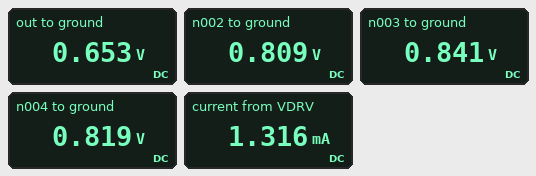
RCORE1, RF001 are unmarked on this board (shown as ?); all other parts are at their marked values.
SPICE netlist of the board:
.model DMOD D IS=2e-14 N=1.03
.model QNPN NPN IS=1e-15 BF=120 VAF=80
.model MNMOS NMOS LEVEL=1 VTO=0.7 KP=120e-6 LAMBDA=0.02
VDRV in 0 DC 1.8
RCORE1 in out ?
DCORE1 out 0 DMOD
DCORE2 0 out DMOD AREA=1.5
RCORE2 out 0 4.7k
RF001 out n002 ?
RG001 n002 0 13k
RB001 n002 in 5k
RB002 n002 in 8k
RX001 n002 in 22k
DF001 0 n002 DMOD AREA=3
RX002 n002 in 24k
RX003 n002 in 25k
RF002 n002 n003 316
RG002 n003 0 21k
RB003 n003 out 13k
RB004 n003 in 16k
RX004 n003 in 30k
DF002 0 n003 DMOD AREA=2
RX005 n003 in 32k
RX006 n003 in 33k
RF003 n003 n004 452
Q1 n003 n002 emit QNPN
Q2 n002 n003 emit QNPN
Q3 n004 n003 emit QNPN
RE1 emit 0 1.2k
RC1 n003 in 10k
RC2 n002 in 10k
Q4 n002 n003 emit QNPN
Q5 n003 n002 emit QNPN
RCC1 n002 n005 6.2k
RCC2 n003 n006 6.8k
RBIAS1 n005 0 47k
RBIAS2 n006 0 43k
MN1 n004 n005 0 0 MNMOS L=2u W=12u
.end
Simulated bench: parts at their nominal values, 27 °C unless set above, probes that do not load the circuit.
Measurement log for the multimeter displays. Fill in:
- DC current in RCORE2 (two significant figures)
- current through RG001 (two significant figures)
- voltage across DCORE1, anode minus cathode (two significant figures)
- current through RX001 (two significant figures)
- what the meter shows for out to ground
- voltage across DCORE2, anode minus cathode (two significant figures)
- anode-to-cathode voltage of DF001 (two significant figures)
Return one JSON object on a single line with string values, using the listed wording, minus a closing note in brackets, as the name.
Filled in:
{"DC current in RCORE2": "140 µA", "current through RG001": "62 µA", "voltage across DCORE1, anode minus cathode": "650 mV", "current through RX001": "45 µA", "what the meter shows for out to ground": "0.653 V", "voltage across DCORE2, anode minus cathode": "-650 mV", "anode-to-cathode voltage of DF001": "-810 mV"}
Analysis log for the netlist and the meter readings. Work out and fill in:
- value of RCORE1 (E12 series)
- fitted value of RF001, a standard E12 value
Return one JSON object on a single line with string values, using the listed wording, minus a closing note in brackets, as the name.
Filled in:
{"value of RCORE1": "2.2 kΩ", "fitted value of RF001, a standard E12 value": "330 Ω"}
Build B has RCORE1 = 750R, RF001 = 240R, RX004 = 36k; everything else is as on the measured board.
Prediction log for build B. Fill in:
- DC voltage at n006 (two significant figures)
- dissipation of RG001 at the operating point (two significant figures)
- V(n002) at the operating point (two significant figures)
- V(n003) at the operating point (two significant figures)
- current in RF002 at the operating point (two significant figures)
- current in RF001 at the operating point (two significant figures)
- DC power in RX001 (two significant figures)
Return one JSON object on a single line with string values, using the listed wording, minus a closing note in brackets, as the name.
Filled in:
{"DC voltage at n006": "710 mV", "dissipation of RG001 at the operating point": "48 µW", "V(n002) at the operating point": "790 mV", "V(n003) at the operating point": "830 mV", "current in RF002 at the operating point": "110 µA", "current in RF001 at the operating point": "500 µA", "DC power in RX001": "46 µW"}
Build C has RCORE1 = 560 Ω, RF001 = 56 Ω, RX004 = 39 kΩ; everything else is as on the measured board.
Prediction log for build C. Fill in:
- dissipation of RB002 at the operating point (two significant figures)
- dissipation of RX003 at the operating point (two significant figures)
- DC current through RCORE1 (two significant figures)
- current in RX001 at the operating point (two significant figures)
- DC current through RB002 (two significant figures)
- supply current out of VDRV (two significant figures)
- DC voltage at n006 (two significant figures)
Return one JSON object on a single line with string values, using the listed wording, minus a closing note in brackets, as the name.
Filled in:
{"dissipation of RB002 at the operating point": "150 µW", "dissipation of RX003 at the operating point": "47 µW", "DC current through RCORE1": "2.0 mA", "current in RX001 at the operating point": "49 µA", "DC current through RB002": "140 µA", "supply current out of VDRV": "2.9 mA", "DC voltage at n006": "660 mV"}
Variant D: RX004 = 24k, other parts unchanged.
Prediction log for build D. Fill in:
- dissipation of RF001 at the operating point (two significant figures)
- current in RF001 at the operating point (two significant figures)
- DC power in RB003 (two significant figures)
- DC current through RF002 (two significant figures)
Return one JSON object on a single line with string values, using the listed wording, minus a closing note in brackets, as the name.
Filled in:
{"dissipation of RF001 at the operating point": "75 µW", "current in RF001 at the operating point": "480 µA", "DC power in RB003": "2.8 µW", "DC current through RF002": "110 µA"}
